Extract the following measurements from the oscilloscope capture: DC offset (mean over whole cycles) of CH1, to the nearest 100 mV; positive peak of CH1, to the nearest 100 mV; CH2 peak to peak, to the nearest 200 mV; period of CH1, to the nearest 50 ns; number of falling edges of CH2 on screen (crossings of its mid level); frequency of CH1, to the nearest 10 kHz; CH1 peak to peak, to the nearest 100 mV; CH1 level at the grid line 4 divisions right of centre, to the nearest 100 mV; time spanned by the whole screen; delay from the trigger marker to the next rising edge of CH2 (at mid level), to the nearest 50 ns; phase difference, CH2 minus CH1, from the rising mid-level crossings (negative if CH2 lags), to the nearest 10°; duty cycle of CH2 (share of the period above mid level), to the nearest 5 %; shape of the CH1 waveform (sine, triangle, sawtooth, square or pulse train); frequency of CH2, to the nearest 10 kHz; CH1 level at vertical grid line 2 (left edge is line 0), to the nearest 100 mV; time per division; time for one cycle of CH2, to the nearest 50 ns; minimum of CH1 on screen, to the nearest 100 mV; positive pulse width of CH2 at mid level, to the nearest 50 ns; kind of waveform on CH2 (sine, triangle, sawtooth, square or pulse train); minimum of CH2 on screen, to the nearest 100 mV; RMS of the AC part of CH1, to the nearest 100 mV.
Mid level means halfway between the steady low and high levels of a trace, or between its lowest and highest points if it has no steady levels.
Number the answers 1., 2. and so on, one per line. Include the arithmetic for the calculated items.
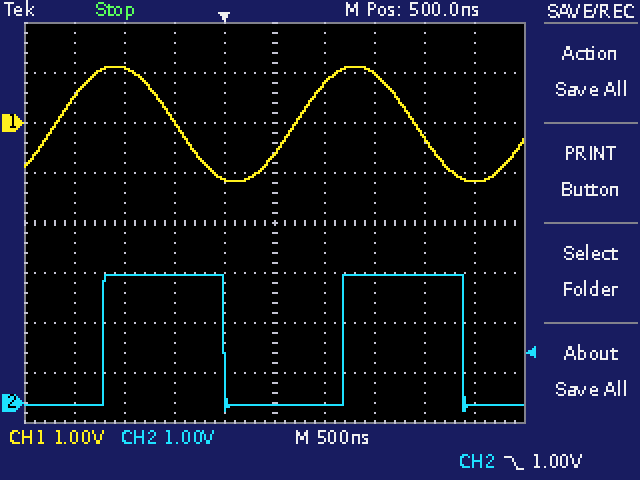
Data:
1. (1.1 V + (-1.2 V)) / 2 ≈ 0.0 V
2. 1.1 V
3. 2.8 V
4. 2.40 µs
5. 2
6. 1 / 2.40 µs ≈ 417 kHz, so 420 kHz to the nearest 10 kHz
7. 1.1 V − (-1.2 V) = 2.3 V
8. -1.2 V
9. 5 µs
10. 1.20 µs
11. -70°
12. 1.20 µs / 2.40 µs ≈ 50 %
13. sine
14. 1 / 2.40 µs ≈ 417 kHz, so 420 kHz to the nearest 10 kHz
15. 1.1 V
16. 500 ns
17. 2.40 µs
18. -1.2 V
19. 1.20 µs
20. square
21. -200 mV
22. 2.3 V / (2√2) ≈ 813 mV, so 800 mV to the nearest 100 mV
